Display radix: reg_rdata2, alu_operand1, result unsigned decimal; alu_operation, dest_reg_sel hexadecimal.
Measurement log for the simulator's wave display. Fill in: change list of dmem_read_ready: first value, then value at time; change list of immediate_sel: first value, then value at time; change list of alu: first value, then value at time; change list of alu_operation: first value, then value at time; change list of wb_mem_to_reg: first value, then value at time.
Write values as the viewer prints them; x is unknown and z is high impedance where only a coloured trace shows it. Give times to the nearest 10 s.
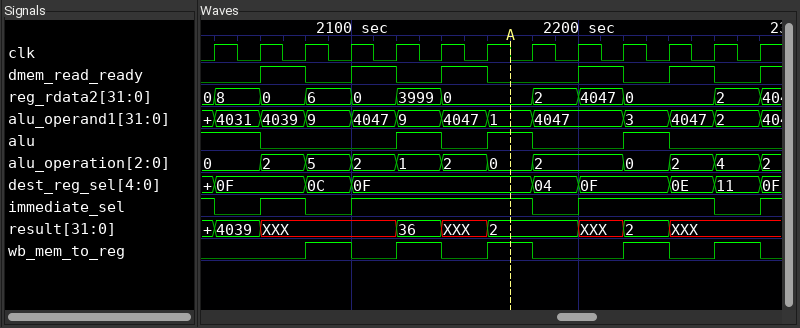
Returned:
0, 1 at 2060 s, 0 at 2080 s, 1 at 2100 s, 0 at 2120 s, 1 at 2140 s, 0 at 2160 s, 1 at 2200 s, 0 at 2220 s, 1 at 2240 s, 0 at 2260 s, 1 at 2280 s
1, 0 at 2040 s, 1 at 2060 s, 0 at 2080 s, 1 at 2100 s, 0 at 2180 s, 1 at 2200 s, 0 at 2260 s, 1 at 2280 s
1, 0 at 2060 s, 1 at 2120 s, 0 at 2140 s, 1 at 2160 s, 0 at 2180 s, 1 at 2220 s, 0 at 2240 s
0, 2 at 2060 s, 5 at 2080 s, 2 at 2100 s, 1 at 2120 s, 2 at 2140 s, 0 at 2160 s, 2 at 2180 s, 0 at 2220 s, 2 at 2240 s, 4 at 2260 s, 2 at 2280 s
0, 1 at 2080 s, 0 at 2100 s, 1 at 2120 s, 0 at 2140 s, 1 at 2160 s, 0 at 2180 s, 1 at 2220 s, 0 at 2240 s, 1 at 2260 s, 0 at 2280 s
